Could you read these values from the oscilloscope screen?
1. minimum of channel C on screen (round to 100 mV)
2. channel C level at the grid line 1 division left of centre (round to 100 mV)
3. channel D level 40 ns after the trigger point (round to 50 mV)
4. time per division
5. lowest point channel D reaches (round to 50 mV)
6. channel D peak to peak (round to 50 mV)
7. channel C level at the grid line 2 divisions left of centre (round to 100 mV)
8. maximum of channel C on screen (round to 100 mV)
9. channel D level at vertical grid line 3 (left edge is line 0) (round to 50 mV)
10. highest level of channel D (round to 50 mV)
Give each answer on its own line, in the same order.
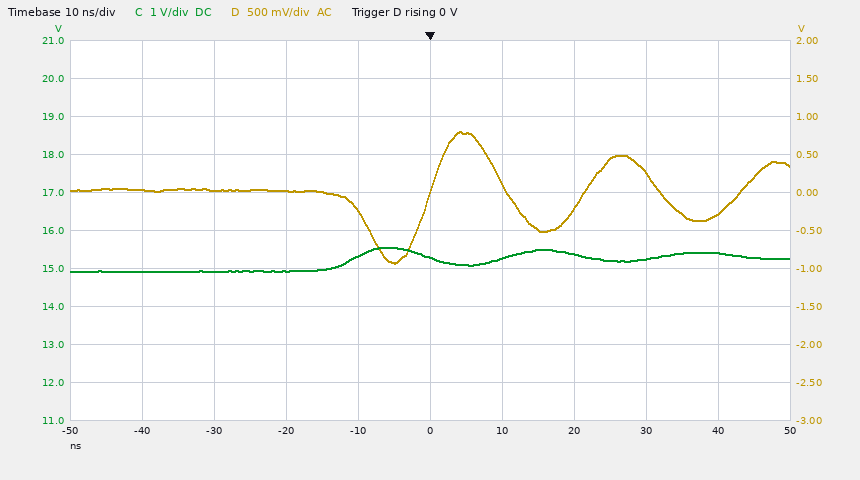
14.9 V
15.3 V
-300 mV
10 ns
-950 mV
1.75 V
14.9 V
15.6 V
0 mV
800 mV
